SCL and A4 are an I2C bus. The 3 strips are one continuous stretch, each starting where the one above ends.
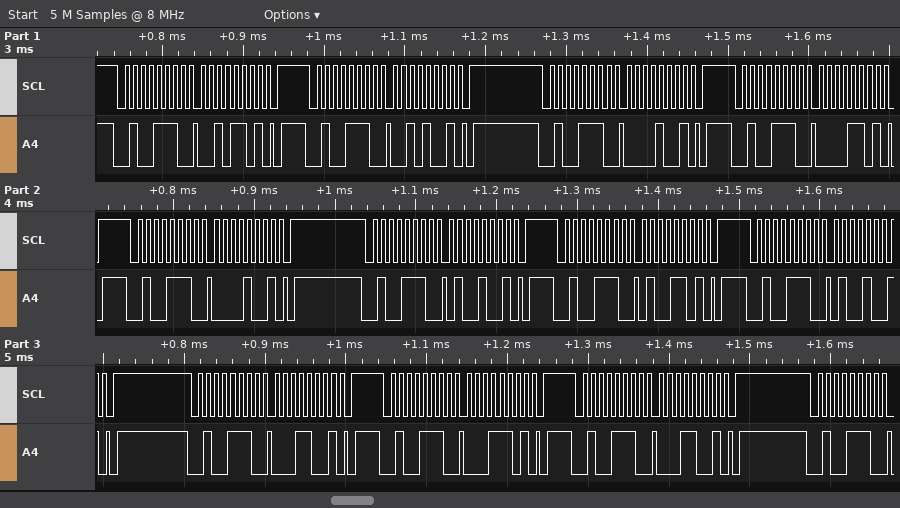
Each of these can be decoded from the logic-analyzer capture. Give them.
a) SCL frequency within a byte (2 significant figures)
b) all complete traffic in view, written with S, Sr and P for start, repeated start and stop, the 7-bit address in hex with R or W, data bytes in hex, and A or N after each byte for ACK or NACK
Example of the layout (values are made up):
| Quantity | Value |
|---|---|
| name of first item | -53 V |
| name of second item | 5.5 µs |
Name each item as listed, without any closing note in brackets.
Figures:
| Quantity | Value |
|---|---|
| SCL frequency within a byte | 100 kHz |
| all complete traffic in view, written with S, Sr and P for start, repeated start and stop, the 7-bit address in hex with R or W, data bytes in hex, and A or N after each byte for ACK or NACK | S 27W A 2D A P S 27W A 29 A P S 27W A 09 A P S 27W A 0D A P S 27W A 09 A P S 27W A 49 A P S 27W A 4D A P S 27W A 49 A P S 27W A 19 A P S 27W A 1D A P S 27W A 19 A P S 27W A |
